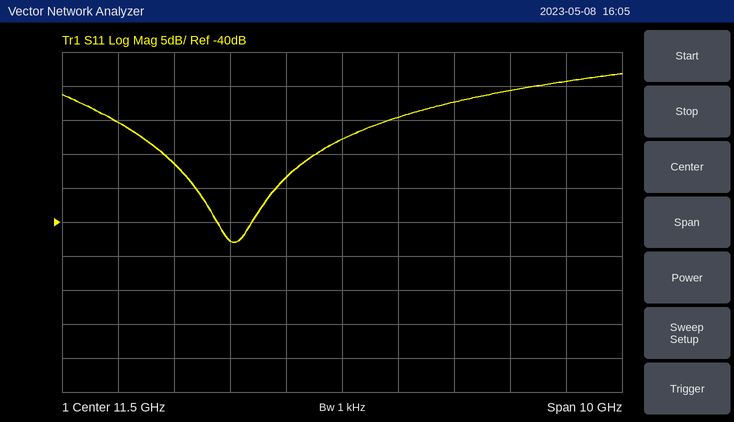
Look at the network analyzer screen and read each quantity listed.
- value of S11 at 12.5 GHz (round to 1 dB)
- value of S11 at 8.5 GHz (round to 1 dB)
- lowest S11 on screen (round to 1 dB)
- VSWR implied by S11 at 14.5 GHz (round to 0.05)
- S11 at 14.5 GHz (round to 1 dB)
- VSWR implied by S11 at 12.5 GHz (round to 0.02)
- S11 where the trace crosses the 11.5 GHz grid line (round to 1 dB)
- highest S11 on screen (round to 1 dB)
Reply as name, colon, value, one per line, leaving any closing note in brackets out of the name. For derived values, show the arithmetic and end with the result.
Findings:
value of S11 at 12.5 GHz: -25 dB
value of S11 at 8.5 GHz: -31 dB
lowest S11 on screen: -43 dB
VSWR implied by S11 at 14.5 GHz: |Γ| = 10^(-21/20) = 0.0891; VSWR = (1 + 0.0891)/(1 − 0.0891) ≈ 1.20
S11 at 14.5 GHz: -21 dB
VSWR implied by S11 at 12.5 GHz: |Γ| = 10^(-25/20) = 0.0562; VSWR = (1 + 0.0562)/(1 − 0.0562) ≈ 1.12
S11 where the trace crosses the 11.5 GHz grid line: -28 dB
highest S11 on screen: -18 dB
